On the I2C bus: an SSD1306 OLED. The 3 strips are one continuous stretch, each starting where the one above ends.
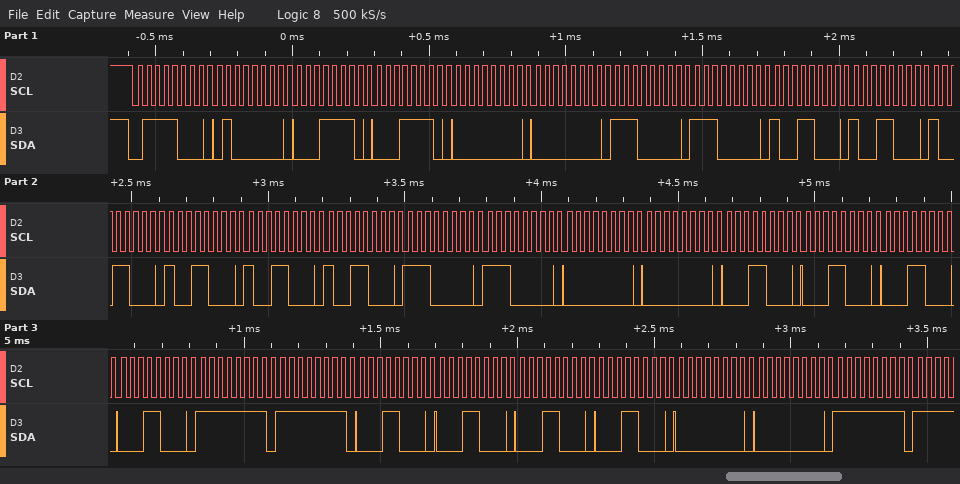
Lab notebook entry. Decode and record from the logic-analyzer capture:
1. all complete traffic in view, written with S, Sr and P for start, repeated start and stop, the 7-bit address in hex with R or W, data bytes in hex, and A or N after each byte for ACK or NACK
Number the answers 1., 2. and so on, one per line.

1. S 3CW A 40 A 1E A 1E A 00 A 00 A E0 A E0 A 98 A 98 A 98 A 98 A 98 A 98 A E0 A E0 A 00 A 00 A 18 A 18 A 18 A 18 A FF A FF A 18 A 18 A 18 A 18 A 00 A 00 A FF A
